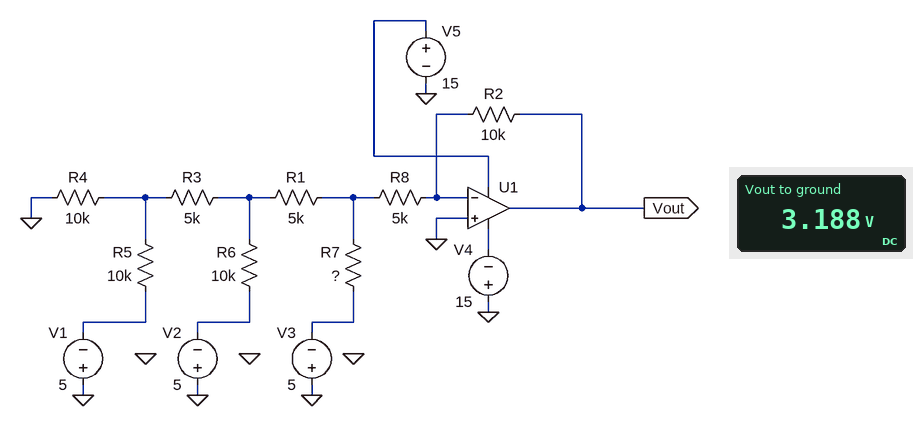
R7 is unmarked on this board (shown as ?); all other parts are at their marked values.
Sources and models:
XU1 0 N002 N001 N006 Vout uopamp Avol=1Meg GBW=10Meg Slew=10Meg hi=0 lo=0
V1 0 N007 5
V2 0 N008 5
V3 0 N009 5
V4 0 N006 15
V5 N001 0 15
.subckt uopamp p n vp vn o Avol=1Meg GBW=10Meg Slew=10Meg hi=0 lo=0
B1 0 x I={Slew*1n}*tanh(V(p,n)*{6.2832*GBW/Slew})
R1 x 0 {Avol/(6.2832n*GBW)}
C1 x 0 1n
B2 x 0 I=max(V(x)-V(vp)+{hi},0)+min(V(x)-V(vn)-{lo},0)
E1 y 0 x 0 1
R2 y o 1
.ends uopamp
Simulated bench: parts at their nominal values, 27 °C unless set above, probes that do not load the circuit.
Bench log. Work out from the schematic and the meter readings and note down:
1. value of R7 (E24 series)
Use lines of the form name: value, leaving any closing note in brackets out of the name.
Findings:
value of R7: 33 kΩ
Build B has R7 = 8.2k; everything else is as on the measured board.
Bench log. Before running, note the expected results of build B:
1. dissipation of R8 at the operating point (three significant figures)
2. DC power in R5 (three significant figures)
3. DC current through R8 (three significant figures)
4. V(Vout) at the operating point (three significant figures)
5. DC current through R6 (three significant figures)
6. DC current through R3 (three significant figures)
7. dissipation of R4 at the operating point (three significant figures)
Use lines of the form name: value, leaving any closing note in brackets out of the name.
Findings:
dissipation of R8 at the operating point: 1.09 mW
DC power in R5: 497 µW
DC current through R8: 467 µA
V(Vout) at the operating point: 4.67 V
DC current through R6: 196 µA
DC current through R3: 54.2 µA
dissipation of R4 at the operating point: 768 µW
